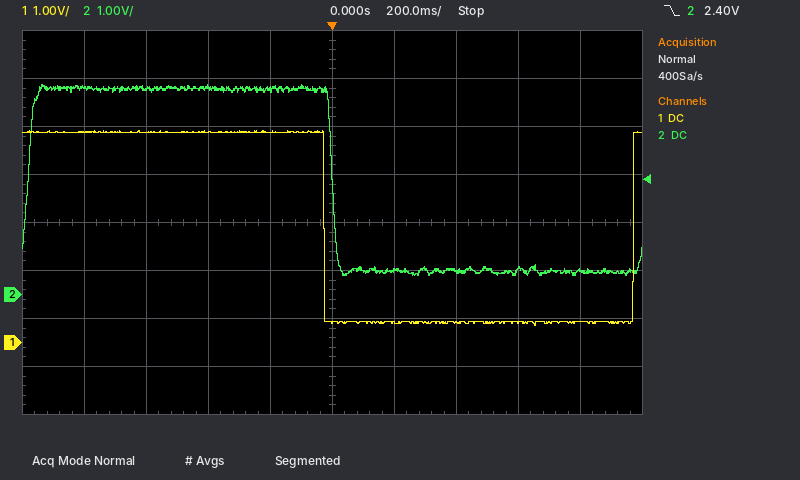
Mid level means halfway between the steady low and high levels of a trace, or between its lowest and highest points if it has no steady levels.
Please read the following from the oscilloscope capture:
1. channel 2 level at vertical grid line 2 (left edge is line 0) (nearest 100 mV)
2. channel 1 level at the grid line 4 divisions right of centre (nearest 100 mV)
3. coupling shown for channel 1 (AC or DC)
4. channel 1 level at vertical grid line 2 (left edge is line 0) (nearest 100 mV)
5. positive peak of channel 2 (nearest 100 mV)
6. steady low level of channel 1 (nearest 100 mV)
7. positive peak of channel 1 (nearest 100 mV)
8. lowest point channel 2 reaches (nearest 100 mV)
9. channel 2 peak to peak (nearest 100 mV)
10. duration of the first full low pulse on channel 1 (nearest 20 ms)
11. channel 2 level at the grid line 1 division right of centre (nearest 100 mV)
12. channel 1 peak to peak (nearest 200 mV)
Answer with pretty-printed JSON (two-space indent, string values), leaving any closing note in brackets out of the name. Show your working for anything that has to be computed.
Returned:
{
  "channel 2 level at vertical grid line 2 (left edge is line 0)": "4.3 V",
  "channel 1 level at the grid line 4 divisions right of centre": "400 mV",
  "coupling shown for channel 1": "DC",
  "channel 1 level at vertical grid line 2 (left edge is line 0)": "4.4 V",
  "positive peak of channel 2": "4.4 V",
  "steady low level of channel 1": "400 mV",
  "positive peak of channel 1": "4.4 V",
  "lowest point channel 2 reaches": "400 mV",
  "channel 2 peak to peak": "4.4 V − (400 mV) = 4.0 V",
  "duration of the first full low pulse on channel 1": "1.00 s",
  "channel 2 level at the grid line 1 division right of centre": "500 mV",
  "channel 1 peak to peak": "4.0 V"
}
